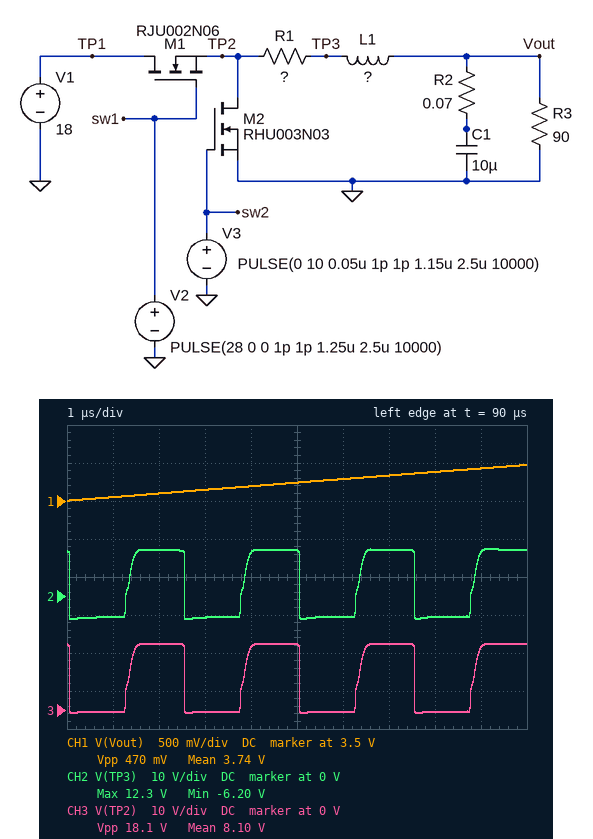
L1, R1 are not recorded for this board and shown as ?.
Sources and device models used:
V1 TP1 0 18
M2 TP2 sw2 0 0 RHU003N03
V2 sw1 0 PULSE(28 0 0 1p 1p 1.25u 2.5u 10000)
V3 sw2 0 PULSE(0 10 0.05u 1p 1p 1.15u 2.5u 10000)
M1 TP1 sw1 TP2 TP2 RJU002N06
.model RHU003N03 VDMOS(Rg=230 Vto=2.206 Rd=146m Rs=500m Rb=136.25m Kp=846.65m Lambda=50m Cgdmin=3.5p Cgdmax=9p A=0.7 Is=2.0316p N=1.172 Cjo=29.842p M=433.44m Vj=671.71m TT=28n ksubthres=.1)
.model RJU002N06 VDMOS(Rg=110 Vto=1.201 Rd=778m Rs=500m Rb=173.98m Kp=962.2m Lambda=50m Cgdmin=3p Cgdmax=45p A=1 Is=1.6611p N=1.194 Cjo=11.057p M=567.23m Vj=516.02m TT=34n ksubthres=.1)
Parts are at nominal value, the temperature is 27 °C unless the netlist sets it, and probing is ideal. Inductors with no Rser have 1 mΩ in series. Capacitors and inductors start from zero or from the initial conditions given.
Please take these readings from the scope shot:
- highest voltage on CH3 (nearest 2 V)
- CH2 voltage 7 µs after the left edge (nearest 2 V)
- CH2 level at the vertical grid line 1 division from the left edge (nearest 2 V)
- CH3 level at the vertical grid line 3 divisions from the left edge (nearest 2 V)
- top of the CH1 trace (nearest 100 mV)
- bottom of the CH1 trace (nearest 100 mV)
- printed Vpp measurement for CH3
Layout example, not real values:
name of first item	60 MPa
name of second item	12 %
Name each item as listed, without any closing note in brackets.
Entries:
highest voltage on CH3	18 V
CH2 voltage 7 µs after the left edge	12 V
CH2 level at the vertical grid line 1 division from the left edge	-6 V
CH3 level at the vertical grid line 3 divisions from the left edge	0 V
top of the CH1 trace	4.0 V
bottom of the CH1 trace	3.5 V
printed Vpp measurement for CH3	18.1 V
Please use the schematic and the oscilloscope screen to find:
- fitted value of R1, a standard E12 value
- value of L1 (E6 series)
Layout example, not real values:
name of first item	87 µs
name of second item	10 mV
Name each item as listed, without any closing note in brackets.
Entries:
fitted value of R1, a standard E12 value	10 Ω
value of L1	470 µH
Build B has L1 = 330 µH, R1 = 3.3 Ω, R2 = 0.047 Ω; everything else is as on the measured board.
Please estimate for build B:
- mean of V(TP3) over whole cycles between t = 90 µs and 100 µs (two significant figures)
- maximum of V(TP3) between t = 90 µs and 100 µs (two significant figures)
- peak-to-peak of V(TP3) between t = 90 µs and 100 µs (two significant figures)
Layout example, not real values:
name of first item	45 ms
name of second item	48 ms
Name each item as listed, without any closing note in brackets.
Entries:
mean of V(TP3) over whole cycles between t = 90 µs and 100 µs	4.8 V
maximum of V(TP3) between t = 90 µs and 100 µs	14 V
peak-to-peak of V(TP3) between t = 90 µs and 100 µs	18 V
